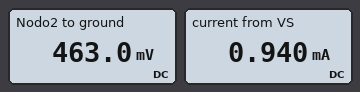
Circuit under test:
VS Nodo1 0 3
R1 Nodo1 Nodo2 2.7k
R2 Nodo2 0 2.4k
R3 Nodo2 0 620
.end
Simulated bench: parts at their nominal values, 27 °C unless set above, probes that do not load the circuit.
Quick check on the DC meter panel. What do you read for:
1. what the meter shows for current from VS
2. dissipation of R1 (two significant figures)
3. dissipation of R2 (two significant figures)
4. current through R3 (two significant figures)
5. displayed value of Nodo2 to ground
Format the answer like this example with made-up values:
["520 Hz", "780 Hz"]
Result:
["0.940 mA", "2.4 mW", "89 µW", "750 µA", "463.0 mV"]
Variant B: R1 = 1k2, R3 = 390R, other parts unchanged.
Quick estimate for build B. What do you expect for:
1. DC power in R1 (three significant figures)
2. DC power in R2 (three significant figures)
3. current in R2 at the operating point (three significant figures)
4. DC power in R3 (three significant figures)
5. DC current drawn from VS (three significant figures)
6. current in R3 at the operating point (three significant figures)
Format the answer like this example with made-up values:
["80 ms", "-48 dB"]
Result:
["4.58 mW", "179 µW", "273 µA", "1.10 mW", "1.95 mA", "1.68 mA"]
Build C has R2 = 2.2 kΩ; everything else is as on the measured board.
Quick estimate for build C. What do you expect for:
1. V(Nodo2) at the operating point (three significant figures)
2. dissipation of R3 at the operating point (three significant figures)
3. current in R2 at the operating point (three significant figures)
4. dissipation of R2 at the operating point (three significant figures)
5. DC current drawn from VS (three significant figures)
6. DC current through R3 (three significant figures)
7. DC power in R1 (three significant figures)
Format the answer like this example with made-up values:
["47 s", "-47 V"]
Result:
["456 mV", "335 µW", "207 µA", "94.4 µW", "942 µA", "735 µA", "2.40 mW"]
